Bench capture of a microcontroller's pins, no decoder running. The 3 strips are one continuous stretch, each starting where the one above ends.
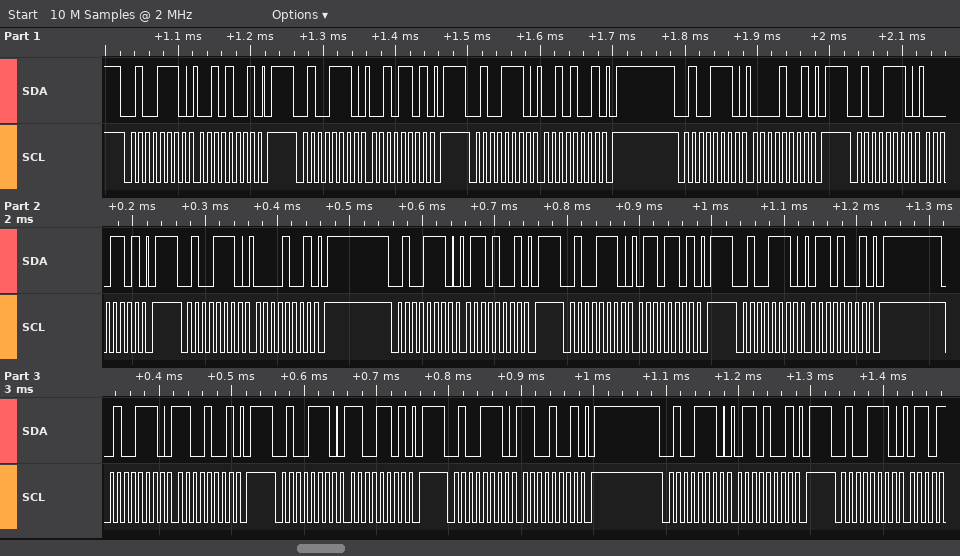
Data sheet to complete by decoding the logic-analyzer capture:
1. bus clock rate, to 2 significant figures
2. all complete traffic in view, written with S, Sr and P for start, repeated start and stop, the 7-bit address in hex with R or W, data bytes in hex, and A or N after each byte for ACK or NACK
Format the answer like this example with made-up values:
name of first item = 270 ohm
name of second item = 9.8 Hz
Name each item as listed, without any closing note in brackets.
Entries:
bus clock rate, to 2 significant figures = 100 kHz
all complete traffic in view, written with S, Sr and P for start, repeated start and stop, the 7-bit address in hex with R or W, data bytes in hex, and A or N after each byte for ACK or NACK = S 27W A 29 A P S 27W A 2D A P S 27W A 29 A P S 27W A 09 A P S 27W A 0D A P S 27W A 09 A P S 27W A 69 A P S 27W A 6D A P S 27W A 69 A P S 27W A C9 A P S 27W A CD A P S 27W A C9 A P S 27W A 69 A P S 27W A
